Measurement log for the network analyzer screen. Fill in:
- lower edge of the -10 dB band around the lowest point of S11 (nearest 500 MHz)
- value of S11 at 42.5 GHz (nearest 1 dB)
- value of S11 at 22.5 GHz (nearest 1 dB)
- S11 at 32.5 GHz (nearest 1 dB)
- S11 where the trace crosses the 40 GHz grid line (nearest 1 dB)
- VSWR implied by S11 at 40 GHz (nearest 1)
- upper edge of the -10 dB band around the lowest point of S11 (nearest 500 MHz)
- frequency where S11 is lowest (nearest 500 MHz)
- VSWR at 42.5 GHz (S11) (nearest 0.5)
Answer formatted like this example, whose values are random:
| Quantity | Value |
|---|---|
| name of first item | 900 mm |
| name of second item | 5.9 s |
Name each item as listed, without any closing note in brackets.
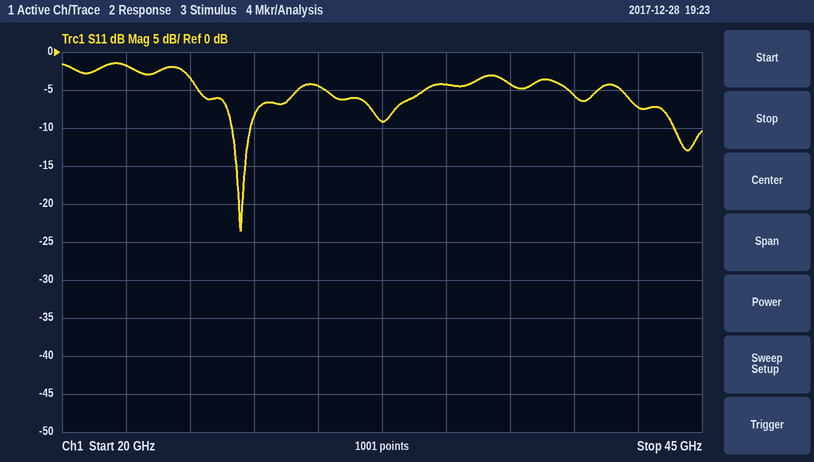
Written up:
| Quantity | Value |
|---|---|
| lower edge of the -10 dB band around the lowest point of S11 | 26.5 GHz |
| value of S11 at 42.5 GHz | -7 dB |
| value of S11 at 22.5 GHz | -2 dB |
| S11 at 32.5 GHz | -9 dB |
| S11 where the trace crosses the 40 GHz grid line | -6 dB |
| VSWR implied by S11 at 40 GHz | 3 |
| upper edge of the -10 dB band around the lowest point of S11 | 27.5 GHz |
| frequency where S11 is lowest | 27.0 GHz |
| VSWR at 42.5 GHz (S11) | 2.5 |
